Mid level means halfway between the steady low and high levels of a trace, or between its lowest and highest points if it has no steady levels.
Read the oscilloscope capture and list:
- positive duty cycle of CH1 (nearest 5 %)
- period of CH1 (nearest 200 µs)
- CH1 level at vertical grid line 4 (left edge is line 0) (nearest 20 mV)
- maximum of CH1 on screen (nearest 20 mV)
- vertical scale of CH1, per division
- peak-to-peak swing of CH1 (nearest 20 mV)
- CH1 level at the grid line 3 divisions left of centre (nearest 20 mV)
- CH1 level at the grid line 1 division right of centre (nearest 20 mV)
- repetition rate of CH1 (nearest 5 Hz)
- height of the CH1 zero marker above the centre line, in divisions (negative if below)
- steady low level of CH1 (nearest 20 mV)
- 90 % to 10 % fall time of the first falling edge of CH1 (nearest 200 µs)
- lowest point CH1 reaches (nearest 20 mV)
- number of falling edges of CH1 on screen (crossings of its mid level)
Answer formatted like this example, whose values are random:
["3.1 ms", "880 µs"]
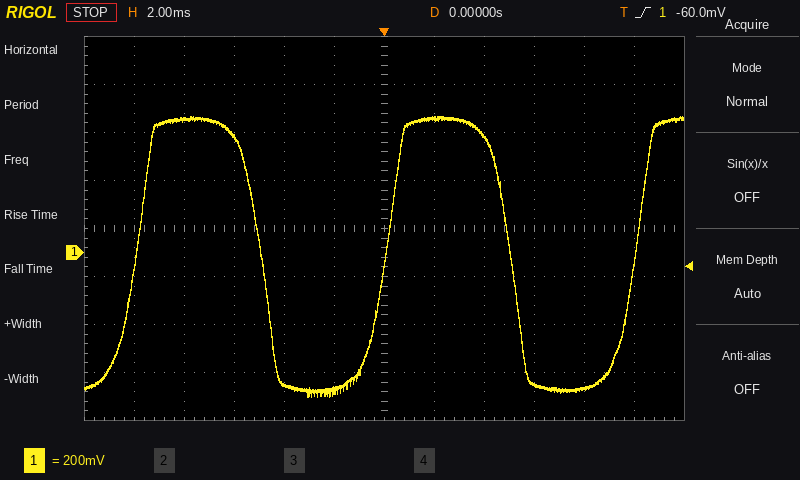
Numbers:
["50 %", "10.0 ms", "-540 mV", "560 mV", "200 mV", "1.16 V", "480 mV", "560 mV", "100 Hz", "-0.5 div", "-560 mV", "1.4 ms", "-600 mV", "2"]
